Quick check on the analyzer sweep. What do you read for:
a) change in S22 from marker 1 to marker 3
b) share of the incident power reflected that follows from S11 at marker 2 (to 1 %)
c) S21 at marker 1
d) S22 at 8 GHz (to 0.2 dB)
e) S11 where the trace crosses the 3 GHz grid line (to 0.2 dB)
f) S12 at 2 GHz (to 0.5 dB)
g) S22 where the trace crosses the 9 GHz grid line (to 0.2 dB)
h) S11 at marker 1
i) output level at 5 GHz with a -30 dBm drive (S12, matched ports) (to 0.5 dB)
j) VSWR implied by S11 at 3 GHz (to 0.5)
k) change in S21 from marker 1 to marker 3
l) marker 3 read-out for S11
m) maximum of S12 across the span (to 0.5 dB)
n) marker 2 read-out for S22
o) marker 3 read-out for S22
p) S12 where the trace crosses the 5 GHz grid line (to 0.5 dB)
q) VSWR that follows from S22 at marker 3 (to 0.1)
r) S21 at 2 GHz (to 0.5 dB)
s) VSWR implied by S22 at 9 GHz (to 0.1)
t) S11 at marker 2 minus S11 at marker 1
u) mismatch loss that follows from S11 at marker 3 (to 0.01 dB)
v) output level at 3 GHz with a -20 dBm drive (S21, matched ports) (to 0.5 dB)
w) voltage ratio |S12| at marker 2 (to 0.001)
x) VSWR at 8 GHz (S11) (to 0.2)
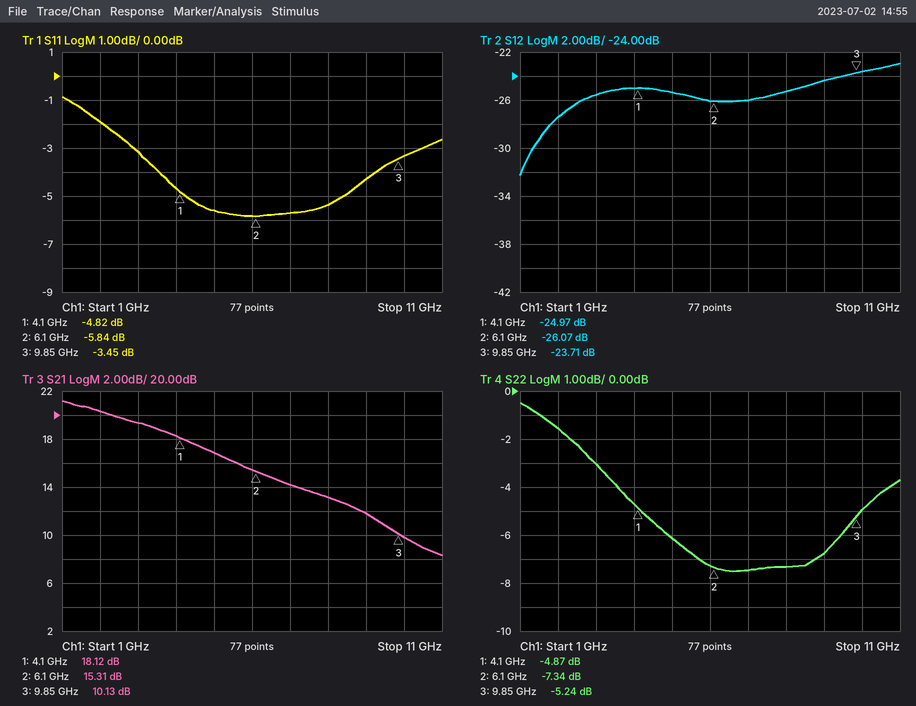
-0.37 dB
26 %
18.12 dB
-7.4 dB
-3.2 dB
-27.5 dB
-6.8 dB
-4.82 dB
-55.5 dBm
5.5
-7.99 dB
-3.45 dB
-23.0 dB
-7.34 dB
-5.24 dB
-25.5 dB
3.4
20.5 dB
2.7
-1.02 dB
2.61 dB
-0.5 dBm
0.050
3.4
